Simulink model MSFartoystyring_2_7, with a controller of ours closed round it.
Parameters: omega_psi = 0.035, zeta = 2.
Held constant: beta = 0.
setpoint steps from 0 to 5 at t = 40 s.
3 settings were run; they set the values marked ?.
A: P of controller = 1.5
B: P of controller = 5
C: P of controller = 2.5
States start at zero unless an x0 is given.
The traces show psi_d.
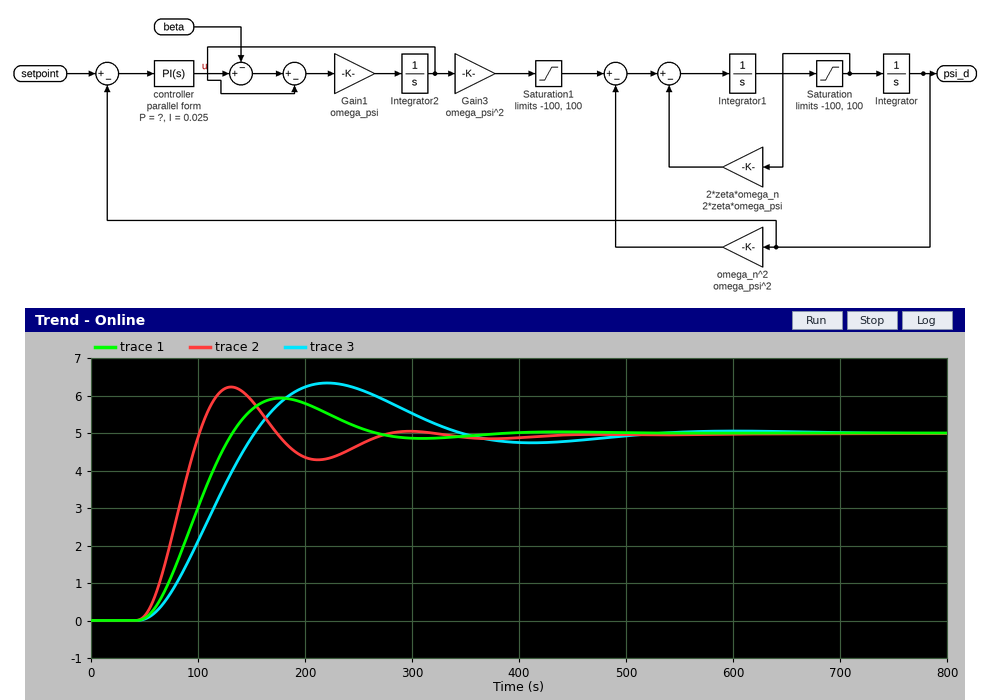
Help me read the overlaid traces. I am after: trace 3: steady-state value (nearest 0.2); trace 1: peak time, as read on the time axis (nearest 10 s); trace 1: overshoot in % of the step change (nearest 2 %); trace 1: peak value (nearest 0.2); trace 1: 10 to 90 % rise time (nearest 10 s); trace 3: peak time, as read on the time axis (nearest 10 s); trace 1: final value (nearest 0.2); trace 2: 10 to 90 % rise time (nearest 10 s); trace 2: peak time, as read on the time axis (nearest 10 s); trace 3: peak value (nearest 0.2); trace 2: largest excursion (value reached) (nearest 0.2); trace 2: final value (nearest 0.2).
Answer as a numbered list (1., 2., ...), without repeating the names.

1. 5.0
2. 180 s
3. 18 %
4. 6.0
5. 60 s
6. 220 s
7. 5.0
8. 40 s
9. 130 s
10. 6.4
11. 6.2
12. 5.0
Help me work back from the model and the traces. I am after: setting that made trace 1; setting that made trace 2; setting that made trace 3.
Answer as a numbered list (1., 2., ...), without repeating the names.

1. C
2. B
3. A
